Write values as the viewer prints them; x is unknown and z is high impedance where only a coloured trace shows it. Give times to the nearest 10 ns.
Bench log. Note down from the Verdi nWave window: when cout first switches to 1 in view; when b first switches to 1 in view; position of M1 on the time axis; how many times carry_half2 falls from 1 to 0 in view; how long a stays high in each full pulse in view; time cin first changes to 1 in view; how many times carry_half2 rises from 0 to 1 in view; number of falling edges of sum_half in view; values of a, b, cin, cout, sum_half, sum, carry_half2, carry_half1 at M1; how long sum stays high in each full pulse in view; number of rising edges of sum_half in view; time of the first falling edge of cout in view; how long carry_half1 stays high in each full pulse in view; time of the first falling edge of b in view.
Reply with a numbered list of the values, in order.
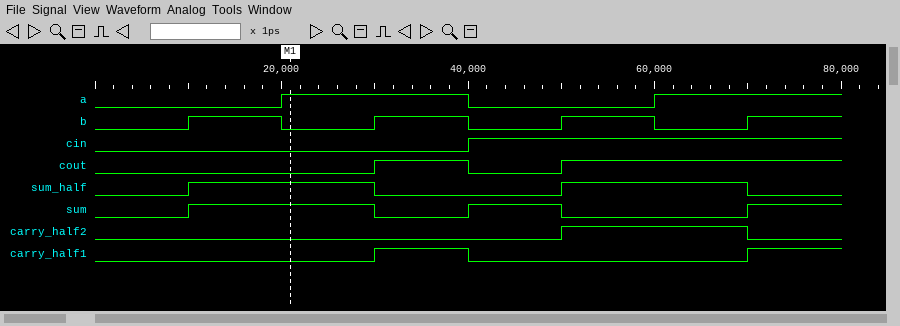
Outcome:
1. 30 ns
2. 10 ns
3. 20 ns
4. 1
5. 20 ns
6. 40 ns
7. 1
8. 2
9. a=1, b=0, cin=0, cout=0, sum_half=1, sum=1, carry_half2=0, carry_half1=0
10. 20 ns, 10 ns
11. 2
12. 40 ns
13. 10 ns
14. 20 ns
